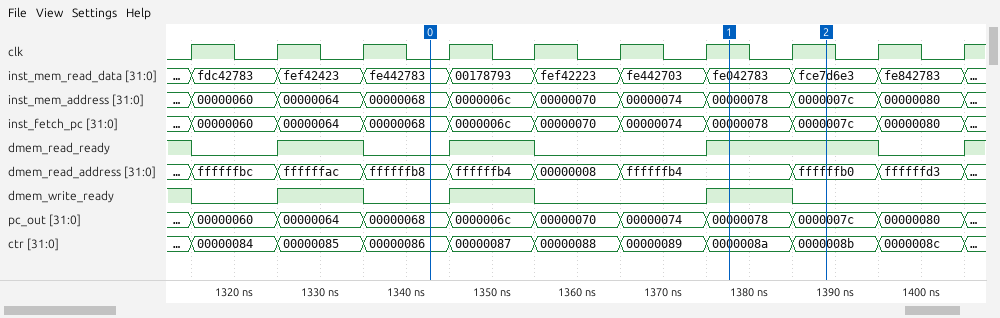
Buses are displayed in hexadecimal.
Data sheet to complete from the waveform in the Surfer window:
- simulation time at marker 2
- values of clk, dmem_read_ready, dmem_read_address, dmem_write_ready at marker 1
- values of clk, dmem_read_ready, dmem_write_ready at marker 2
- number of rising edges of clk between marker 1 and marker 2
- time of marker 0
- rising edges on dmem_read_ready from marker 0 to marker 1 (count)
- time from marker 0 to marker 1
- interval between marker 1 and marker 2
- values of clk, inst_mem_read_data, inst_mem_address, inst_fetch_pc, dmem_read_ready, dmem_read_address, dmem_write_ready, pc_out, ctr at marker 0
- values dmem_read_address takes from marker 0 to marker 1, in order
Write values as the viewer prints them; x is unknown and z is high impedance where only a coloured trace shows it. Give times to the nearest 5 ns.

1390 ns
clk=1, dmem_read_ready=1, dmem_read_address=ffffffb4, dmem_write_ready=1
clk=1, dmem_read_ready=1, dmem_write_ready=0
1
1345 ns
2
35 ns
10 ns
clk=0, inst_mem_read_data=fe442783, inst_mem_address=00000068, inst_fetch_pc=00000068, dmem_read_ready=0, dmem_read_address=ffffffb8, dmem_write_ready=0, pc_out=00000068, ctr=00000086
ffffffb8, ffffffb4, 00000008, ffffffb4
